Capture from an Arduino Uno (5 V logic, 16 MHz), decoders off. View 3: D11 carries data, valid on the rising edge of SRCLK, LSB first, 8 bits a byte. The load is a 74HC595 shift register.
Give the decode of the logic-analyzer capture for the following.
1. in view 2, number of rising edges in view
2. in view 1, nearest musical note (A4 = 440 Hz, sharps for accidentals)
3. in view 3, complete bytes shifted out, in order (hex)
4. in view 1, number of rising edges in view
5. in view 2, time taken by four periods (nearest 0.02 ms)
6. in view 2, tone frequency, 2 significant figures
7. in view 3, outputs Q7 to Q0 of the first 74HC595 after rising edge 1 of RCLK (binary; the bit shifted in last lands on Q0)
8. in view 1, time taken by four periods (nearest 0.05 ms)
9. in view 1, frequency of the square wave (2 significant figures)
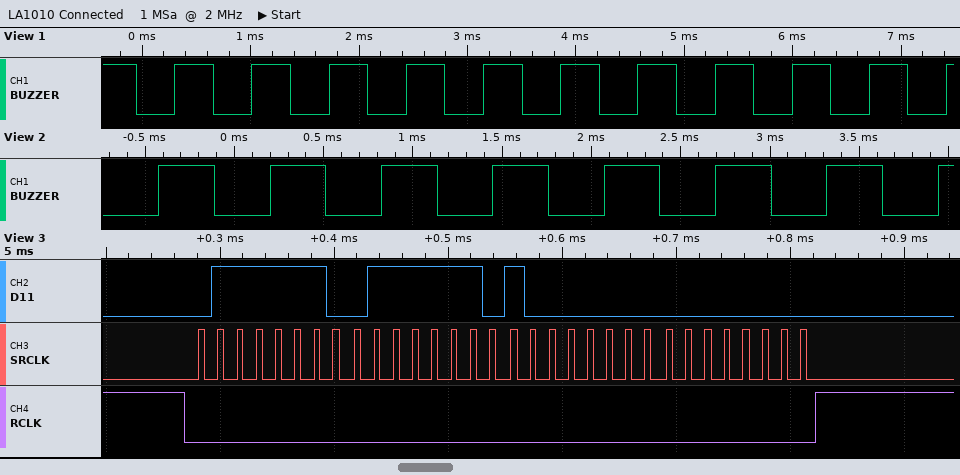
8
F6
7E 7E 01 00
11
2.50 ms
1.6 kHz
00000000
2.85 ms
1.4 kHz
